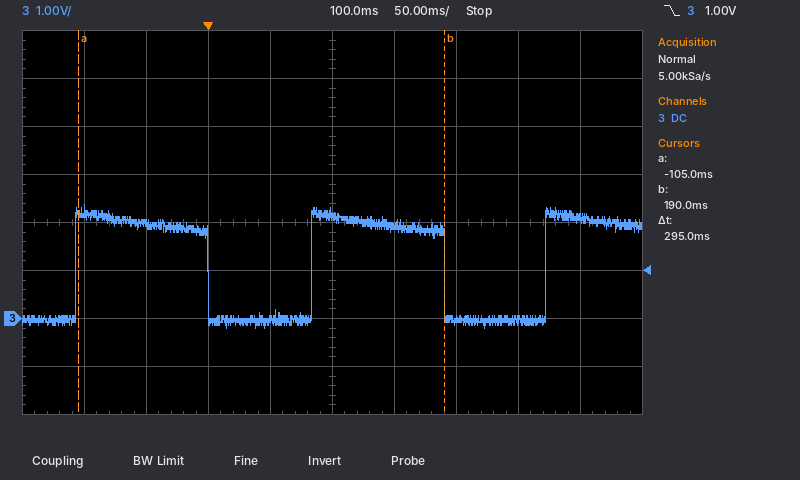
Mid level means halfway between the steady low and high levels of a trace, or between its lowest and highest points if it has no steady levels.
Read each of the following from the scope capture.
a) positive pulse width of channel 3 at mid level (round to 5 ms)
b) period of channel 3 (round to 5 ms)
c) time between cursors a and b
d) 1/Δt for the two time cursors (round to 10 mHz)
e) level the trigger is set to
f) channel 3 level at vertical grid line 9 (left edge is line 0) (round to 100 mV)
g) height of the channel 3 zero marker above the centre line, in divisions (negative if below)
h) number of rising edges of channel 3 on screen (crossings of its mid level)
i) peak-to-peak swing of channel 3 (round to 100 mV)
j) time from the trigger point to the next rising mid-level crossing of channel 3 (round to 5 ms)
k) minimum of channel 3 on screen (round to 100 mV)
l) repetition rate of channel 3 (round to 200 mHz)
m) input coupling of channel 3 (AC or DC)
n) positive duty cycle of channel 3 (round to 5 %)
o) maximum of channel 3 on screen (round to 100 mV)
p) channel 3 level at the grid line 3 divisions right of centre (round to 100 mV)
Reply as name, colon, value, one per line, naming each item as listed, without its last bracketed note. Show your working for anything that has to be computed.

positive pulse width of channel 3 at mid level: 105 ms
period of channel 3: 190 ms
time between cursors a and b: 295 ms
1/Δt for the two time cursors: 1 / 295 ms ≈ 3.39 Hz
level the trigger is set to: 1.00 V
channel 3 level at vertical grid line 9 (left edge is line 0): 2.1 V
height of the channel 3 zero marker above the centre line, in divisions: -2.0 div
number of rising edges of channel 3 on screen: 3
peak-to-peak swing of channel 3: 2.4 V − (-200 mV) = 2.6 V
time from the trigger point to the next rising mid-level crossing of channel 3: 85 ms
minimum of channel 3 on screen: -200 mV
repetition rate of channel 3: 1 / 190 ms ≈ 5.26 Hz, so 5.2 Hz to the nearest 200 mHz
input coupling of channel 3: DC
positive duty cycle of channel 3: 105 ms / 190 ms ≈ 55 %
maximum of channel 3 on screen: 2.4 V
channel 3 level at the grid line 3 divisions right of centre: 0.0 V
